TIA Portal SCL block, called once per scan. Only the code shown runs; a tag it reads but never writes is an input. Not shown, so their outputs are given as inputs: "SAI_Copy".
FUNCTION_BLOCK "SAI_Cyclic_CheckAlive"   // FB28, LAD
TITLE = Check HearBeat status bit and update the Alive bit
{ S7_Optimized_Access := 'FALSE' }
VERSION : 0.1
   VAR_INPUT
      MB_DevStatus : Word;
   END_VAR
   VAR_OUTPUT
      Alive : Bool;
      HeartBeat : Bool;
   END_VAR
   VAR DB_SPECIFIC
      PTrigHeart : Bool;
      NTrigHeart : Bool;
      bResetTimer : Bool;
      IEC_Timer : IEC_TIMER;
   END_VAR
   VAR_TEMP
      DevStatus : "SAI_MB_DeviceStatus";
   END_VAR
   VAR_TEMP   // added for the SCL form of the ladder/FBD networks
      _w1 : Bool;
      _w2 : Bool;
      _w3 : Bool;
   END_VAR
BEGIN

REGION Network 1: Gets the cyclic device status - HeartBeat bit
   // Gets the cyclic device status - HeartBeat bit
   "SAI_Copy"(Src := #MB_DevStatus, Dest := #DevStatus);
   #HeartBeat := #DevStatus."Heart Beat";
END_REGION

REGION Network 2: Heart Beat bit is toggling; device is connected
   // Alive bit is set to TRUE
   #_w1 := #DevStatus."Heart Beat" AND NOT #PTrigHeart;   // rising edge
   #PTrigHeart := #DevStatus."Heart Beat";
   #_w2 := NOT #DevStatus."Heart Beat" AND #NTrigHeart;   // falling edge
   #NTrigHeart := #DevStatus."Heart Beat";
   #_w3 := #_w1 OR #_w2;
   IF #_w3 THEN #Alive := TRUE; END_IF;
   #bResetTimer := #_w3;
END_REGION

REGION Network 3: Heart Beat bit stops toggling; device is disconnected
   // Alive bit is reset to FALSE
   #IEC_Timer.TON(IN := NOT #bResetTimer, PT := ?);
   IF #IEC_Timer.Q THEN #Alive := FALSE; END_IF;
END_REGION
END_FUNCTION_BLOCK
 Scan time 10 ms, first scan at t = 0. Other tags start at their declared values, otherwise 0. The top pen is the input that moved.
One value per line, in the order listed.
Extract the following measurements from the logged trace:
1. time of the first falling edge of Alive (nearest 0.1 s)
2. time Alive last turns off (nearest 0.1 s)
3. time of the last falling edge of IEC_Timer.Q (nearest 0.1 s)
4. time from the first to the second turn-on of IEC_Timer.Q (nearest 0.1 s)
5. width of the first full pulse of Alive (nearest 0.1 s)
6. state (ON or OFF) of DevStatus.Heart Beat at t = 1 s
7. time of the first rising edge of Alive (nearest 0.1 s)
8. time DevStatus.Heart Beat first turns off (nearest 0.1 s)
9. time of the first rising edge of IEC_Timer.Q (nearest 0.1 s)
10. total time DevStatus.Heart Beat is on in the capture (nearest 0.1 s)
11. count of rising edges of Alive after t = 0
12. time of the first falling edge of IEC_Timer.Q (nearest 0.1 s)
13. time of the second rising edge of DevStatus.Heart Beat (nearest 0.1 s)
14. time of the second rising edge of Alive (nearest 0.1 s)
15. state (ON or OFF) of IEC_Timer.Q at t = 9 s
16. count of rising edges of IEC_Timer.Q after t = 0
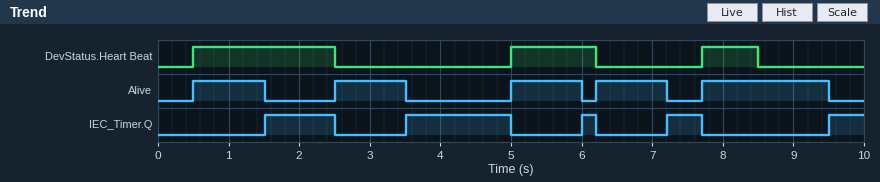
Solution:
1.5 s
9.5 s
7.7 s
2.0 s
1.0 s
ON
0.5 s
2.5 s
1.5 s
4.0 s
5
2.5 s
5.0 s
2.5 s
OFF
5
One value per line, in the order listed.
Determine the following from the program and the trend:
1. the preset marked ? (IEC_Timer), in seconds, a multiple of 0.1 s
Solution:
1.0 s
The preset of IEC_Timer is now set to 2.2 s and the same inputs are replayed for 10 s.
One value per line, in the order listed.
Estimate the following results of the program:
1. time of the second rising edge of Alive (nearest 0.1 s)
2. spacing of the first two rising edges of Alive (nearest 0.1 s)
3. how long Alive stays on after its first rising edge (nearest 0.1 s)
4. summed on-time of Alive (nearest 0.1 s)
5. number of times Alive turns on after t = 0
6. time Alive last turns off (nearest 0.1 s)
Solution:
5.0 s
4.5 s
4.2 s
9.2 s
2
4.7 s
